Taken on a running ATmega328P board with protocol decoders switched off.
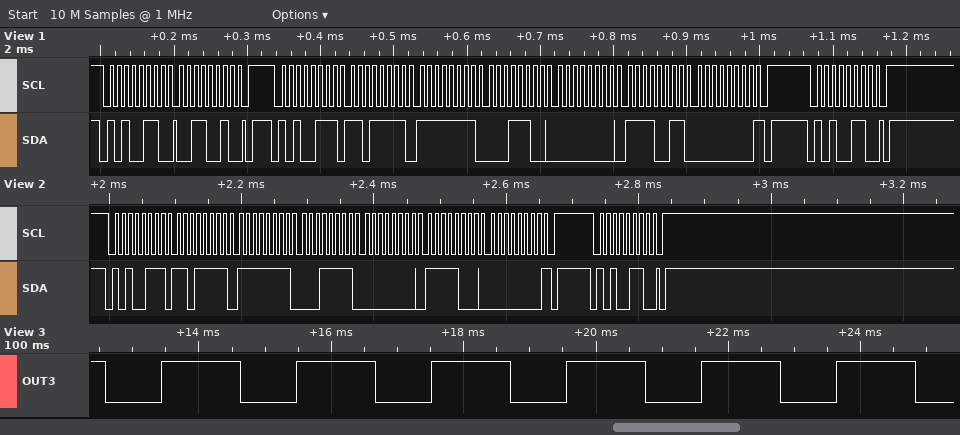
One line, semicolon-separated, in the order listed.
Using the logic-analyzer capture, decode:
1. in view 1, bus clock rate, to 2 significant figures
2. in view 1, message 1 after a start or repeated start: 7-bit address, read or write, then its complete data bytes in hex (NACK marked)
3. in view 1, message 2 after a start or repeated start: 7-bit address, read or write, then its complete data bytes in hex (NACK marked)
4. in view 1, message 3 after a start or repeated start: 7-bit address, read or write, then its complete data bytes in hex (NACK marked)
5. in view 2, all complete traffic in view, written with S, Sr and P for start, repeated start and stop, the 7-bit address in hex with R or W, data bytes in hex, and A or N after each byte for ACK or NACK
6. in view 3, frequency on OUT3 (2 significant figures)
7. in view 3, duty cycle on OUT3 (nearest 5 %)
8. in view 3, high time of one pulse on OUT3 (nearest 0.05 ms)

100 kHz; 0x53 write: 32; 0x53 read: DF FF 1C 00 F3 00 NACK; 0x53 write; S 53R A DF A FF A 1F A 00 A F8 A 00 N P S 53W A P; 490 Hz; 60 %; 1.20 ms
